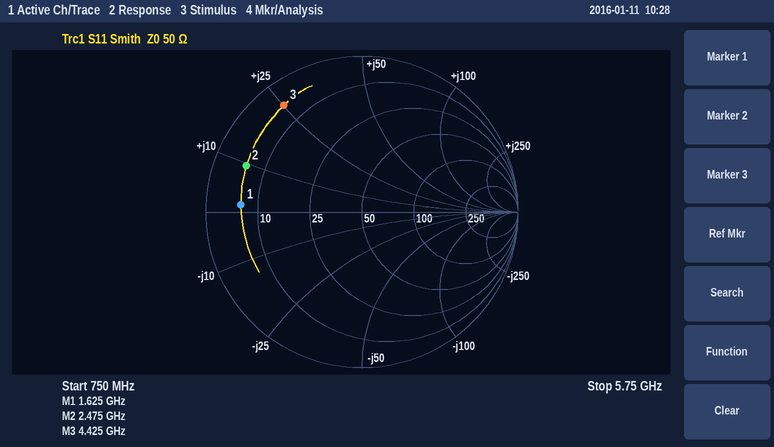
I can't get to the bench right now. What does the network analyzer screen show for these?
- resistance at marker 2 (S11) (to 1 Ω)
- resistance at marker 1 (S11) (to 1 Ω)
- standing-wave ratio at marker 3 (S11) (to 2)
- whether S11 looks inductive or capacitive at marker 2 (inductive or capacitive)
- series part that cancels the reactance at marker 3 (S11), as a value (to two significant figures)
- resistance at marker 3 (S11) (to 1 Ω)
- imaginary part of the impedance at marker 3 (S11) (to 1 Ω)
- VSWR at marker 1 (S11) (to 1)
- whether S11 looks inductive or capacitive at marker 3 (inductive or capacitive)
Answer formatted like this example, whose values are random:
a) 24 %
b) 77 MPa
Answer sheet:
a) 6 Ω
b) 6 Ω
c) 12
d) inductive
e) 1.4 pF
f) 5 Ω
g) +25 Ω
h) 8
i) inductive
